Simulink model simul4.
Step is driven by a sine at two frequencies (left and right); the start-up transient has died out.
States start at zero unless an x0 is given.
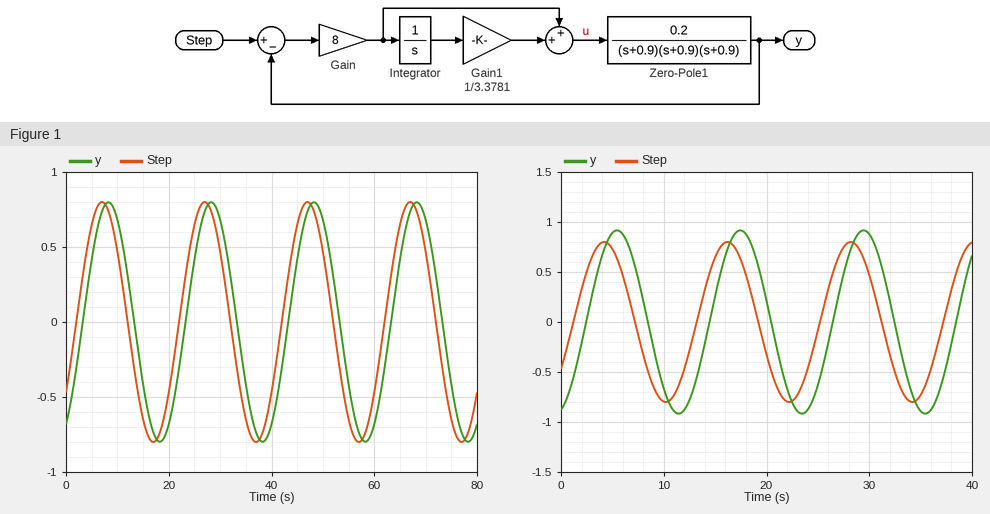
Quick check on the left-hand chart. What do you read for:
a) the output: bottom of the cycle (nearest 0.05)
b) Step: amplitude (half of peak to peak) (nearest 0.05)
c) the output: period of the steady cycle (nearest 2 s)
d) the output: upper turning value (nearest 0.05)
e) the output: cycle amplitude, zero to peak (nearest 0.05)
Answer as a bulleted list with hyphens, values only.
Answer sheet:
- -0.80
- 0.80
- 20 s
- 0.80
- 0.80
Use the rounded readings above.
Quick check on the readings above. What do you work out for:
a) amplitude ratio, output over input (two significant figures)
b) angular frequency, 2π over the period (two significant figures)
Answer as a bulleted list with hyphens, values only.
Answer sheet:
- 1.0
- 0.31 rad/s
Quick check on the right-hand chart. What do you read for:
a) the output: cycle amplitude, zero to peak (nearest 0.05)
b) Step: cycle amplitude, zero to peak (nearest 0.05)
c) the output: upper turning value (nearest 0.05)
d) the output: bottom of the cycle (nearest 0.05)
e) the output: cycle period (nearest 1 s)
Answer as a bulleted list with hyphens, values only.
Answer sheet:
- 0.90
- 0.80
- 0.90
- -0.90
- 12 s
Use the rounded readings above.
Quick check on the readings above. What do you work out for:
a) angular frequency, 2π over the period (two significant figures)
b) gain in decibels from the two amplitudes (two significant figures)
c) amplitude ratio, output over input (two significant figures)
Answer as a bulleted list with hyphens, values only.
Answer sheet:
- 0.52 rad/s
- 1.0 dB
- 1.1
